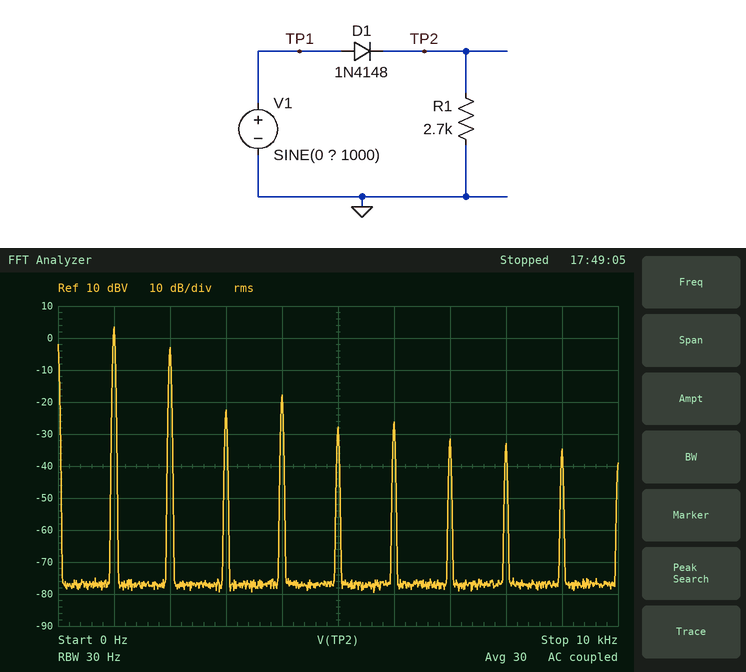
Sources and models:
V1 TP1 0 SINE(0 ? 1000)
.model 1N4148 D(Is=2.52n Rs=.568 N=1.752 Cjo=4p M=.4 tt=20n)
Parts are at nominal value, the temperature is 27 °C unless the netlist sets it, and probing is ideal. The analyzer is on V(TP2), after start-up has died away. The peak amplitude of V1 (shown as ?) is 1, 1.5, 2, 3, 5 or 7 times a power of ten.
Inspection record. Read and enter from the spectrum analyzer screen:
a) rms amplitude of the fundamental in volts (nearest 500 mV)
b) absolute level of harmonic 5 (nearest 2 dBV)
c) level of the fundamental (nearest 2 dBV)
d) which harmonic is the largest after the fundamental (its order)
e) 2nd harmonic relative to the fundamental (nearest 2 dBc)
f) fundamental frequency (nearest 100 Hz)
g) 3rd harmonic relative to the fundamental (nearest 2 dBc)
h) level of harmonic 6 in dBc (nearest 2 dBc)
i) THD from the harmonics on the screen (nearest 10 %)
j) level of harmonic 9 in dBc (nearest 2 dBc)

1.5 V
-28 dBV
4 dBV
2
-6 dBc
1.0 kHz
-26 dBc
-30 dBc
50 %
-38 dBc
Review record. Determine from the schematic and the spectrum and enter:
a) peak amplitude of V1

5 V
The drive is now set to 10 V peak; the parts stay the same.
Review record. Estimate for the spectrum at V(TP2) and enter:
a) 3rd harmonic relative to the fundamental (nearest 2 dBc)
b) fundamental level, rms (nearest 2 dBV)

-32 dBc
10 dBV
